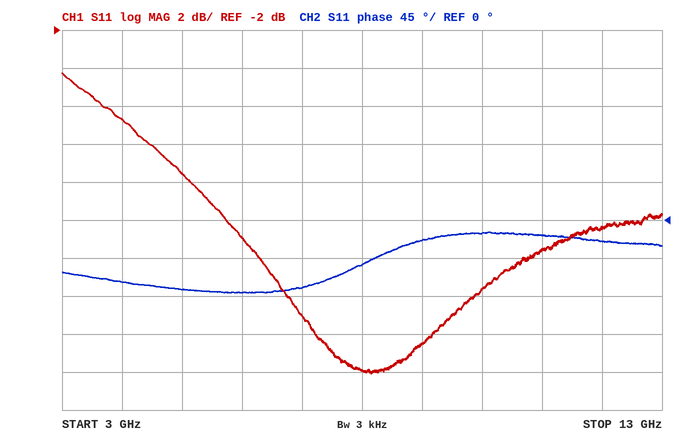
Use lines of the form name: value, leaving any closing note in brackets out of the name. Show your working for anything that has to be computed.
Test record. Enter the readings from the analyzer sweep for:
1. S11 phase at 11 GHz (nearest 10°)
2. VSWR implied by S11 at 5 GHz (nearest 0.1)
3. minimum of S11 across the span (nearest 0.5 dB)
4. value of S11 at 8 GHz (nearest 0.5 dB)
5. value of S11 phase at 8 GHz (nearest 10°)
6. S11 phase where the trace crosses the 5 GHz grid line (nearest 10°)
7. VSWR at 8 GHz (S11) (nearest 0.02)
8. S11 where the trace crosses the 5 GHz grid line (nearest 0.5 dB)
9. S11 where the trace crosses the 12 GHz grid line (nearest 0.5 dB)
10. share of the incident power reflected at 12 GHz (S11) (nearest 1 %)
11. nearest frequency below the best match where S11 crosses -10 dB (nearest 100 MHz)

S11 phase at 11 GHz: -20°
VSWR implied by S11 at 5 GHz: |Γ| = 10^(-9.5/20) = 0.3350; VSWR = (1 + 0.3350)/(1 − 0.3350) ≈ 2.0
minimum of S11 across the span: -20.0 dB
value of S11 at 8 GHz: -20.0 dB
value of S11 phase at 8 GHz: -50°
S11 phase where the trace crosses the 5 GHz grid line: -80°
VSWR at 8 GHz (S11): |Γ| = 10^(-20/20) = 0.1000; VSWR = (1 + 0.1000)/(1 − 0.1000) ≈ 1.22
S11 where the trace crosses the 5 GHz grid line: -9.5 dB
S11 where the trace crosses the 12 GHz grid line: -12.5 dB
share of the incident power reflected at 12 GHz (S11): 10^(-12.5/10) ≈ 6 %
nearest frequency below the best match where S11 crosses -10 dB: 5.1 GHz
